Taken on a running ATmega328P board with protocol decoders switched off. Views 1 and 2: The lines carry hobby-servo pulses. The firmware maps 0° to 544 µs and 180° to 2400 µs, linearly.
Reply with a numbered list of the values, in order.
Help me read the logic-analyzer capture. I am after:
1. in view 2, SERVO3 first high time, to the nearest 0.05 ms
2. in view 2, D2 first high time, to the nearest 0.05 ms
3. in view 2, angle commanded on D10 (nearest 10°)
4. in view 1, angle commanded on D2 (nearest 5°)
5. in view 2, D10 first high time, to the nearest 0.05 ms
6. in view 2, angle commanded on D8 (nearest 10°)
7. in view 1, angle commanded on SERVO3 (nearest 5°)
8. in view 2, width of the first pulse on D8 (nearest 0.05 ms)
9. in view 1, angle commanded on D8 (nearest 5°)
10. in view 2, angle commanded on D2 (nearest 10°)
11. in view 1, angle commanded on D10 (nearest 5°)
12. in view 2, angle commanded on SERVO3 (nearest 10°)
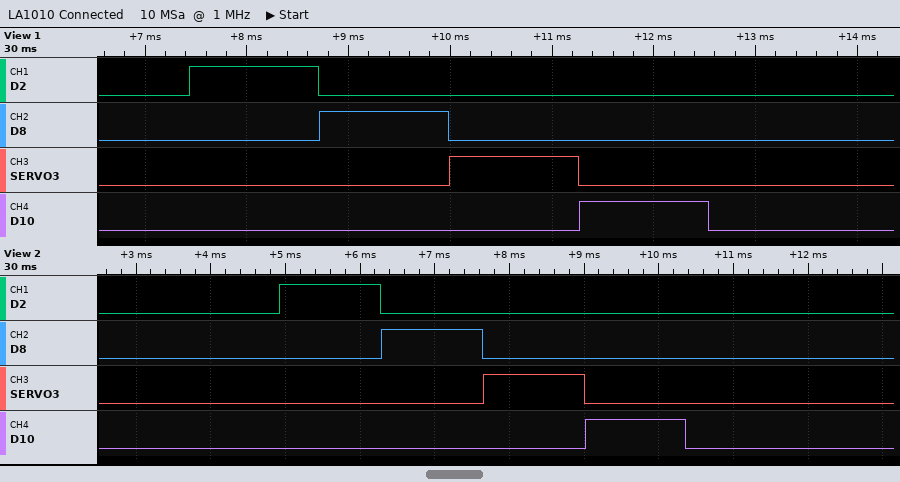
1. 1.35 ms
2. 1.35 ms
3. 80°
4. 70°
5. 1.35 ms
6. 80°
7. 70°
8. 1.35 ms
9. 70°
10. 80°
11. 70°
12. 80°
